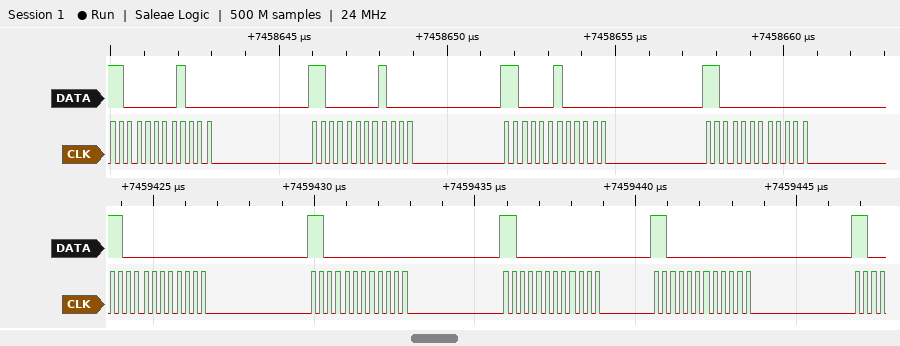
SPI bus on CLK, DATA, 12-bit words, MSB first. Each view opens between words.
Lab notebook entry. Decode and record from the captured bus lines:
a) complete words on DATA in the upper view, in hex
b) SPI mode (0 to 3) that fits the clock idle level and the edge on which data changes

C08, C08, C20, C00
0
